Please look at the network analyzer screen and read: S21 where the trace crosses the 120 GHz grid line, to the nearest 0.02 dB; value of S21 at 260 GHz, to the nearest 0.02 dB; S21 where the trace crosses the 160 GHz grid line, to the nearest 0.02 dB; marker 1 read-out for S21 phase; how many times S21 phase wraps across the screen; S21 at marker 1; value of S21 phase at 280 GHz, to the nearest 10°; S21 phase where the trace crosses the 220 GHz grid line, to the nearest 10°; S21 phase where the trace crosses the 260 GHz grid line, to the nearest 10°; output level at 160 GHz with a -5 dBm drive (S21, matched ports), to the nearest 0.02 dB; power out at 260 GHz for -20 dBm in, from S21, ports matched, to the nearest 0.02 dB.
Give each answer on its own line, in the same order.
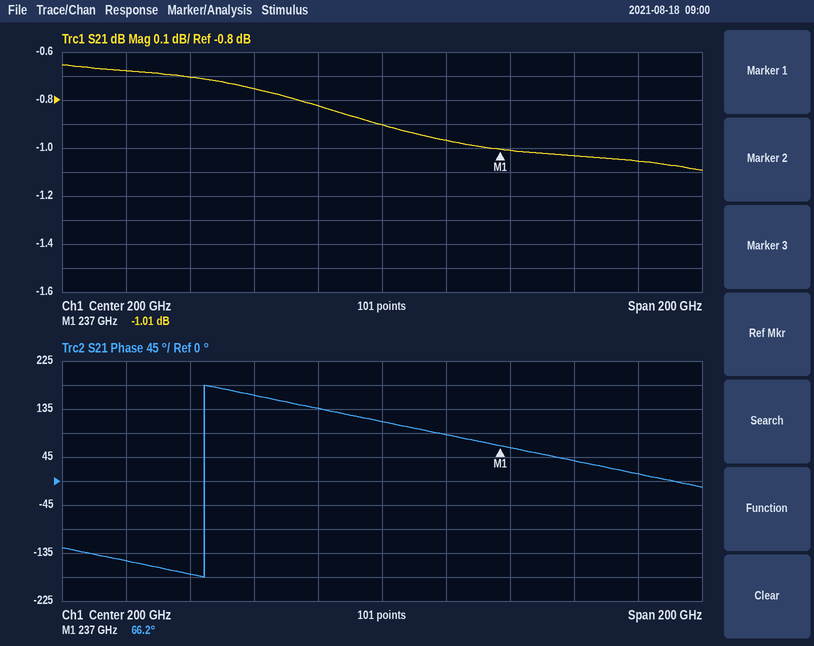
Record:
-0.68 dB
-1.04 dB
-0.76 dB
66.2°
1
-1.01 dB
10°
90°
40°
-5.76 dBm
-21.04 dBm
